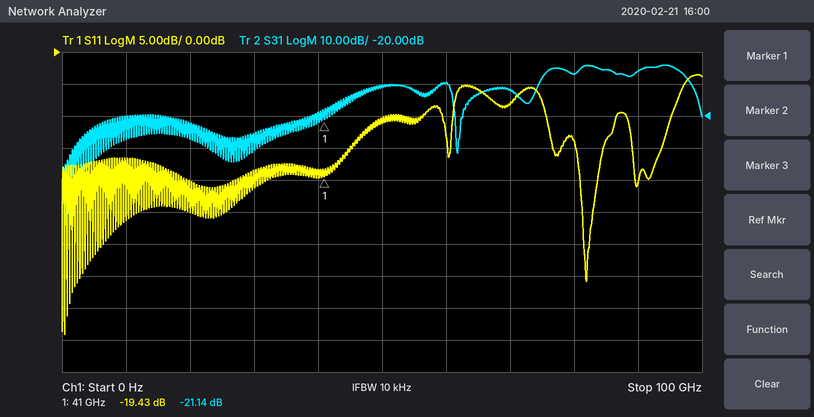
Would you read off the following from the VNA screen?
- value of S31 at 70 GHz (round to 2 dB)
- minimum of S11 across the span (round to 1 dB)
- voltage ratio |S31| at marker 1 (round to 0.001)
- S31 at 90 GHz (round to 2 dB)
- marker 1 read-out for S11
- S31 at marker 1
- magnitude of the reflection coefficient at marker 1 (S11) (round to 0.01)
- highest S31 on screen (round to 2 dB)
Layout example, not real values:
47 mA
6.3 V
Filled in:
-12 dB
-44 dB
0.088
-6 dB
-19.43 dB
-21.14 dB
0.11
-4 dB
